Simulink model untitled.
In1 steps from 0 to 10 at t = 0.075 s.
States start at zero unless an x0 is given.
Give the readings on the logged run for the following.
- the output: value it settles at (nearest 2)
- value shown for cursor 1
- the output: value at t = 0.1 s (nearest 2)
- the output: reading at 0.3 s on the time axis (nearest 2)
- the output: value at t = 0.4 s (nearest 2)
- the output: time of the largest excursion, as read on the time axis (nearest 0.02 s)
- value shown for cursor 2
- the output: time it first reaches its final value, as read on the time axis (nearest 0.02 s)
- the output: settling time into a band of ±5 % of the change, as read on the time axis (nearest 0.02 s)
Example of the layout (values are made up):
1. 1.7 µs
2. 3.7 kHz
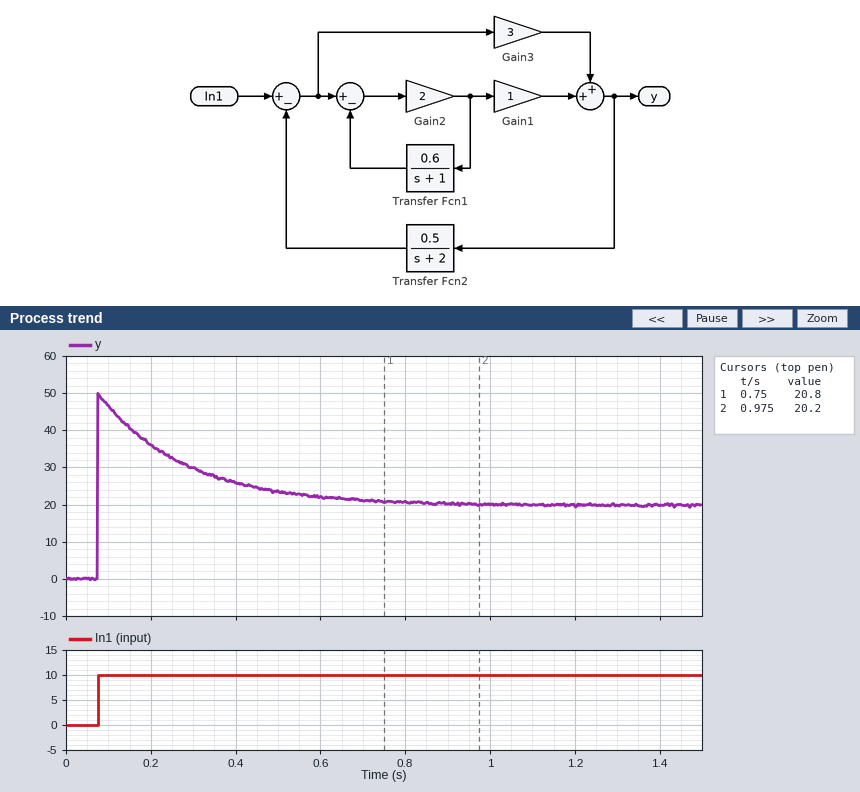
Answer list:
1. 20
2. 20.8
3. 46
4. 30
5. 26
6. 0.08 s
7. 20.2
8. 0.08 s
9. 0.78 s
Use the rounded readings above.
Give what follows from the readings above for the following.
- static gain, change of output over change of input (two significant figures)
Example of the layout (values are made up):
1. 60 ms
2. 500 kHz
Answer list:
1. 2.0
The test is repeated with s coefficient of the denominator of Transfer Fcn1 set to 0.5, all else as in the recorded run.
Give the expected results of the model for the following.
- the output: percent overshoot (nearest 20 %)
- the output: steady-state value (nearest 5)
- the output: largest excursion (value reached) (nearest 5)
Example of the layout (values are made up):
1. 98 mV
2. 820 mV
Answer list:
1. 160 %
2. 20
3. 50
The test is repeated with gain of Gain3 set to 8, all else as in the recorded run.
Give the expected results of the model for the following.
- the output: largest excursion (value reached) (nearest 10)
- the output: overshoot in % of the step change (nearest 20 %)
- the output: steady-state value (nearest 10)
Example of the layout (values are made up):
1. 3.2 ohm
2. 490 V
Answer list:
1. 100
2. 260 %
3. 30
